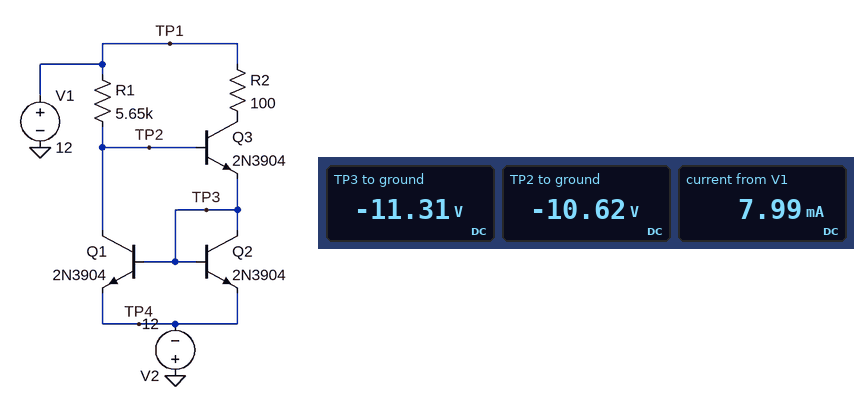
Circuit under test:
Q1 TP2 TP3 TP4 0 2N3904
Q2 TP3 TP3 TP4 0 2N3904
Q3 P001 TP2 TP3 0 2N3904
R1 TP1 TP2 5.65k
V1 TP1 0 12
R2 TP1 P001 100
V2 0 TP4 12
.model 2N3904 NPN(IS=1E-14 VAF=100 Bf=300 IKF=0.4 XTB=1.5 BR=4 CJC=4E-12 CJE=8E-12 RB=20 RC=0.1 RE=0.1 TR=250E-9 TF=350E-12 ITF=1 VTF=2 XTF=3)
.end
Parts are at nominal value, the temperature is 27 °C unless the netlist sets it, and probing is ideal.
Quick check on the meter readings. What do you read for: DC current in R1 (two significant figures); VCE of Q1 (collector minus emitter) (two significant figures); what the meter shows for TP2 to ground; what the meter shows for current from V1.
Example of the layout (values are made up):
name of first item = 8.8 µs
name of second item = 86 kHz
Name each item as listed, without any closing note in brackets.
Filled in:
DC current in R1 = 4.0 mA
VCE of Q1 (collector minus emitter) = 1.4 V
what the meter shows for TP2 to ground = -10.62 V
what the meter shows for current from V1 = 7.99 mA
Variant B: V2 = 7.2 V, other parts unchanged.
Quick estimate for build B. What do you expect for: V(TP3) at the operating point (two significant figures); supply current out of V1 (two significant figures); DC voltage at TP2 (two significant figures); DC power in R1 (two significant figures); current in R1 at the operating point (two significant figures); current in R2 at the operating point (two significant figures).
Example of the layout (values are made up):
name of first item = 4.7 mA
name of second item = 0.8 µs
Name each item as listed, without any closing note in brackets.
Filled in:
V(TP3) at the operating point = -6.5 V
supply current out of V1 = 6.3 mA
DC voltage at TP2 = -5.8 V
DC power in R1 = 56 mW
current in R1 at the operating point = 3.2 mA
current in R2 at the operating point = 3.1 mA
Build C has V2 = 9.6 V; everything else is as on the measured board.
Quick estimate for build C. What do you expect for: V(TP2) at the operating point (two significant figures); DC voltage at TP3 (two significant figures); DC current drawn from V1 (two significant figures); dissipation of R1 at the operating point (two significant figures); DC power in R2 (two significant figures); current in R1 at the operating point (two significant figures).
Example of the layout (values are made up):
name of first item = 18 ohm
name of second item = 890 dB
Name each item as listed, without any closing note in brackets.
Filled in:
V(TP2) at the operating point = -8.2 V
DC voltage at TP3 = -8.9 V
DC current drawn from V1 = 7.1 mA
dissipation of R1 at the operating point = 72 mW
DC power in R2 = 1.3 mW
current in R1 at the operating point = 3.6 mA
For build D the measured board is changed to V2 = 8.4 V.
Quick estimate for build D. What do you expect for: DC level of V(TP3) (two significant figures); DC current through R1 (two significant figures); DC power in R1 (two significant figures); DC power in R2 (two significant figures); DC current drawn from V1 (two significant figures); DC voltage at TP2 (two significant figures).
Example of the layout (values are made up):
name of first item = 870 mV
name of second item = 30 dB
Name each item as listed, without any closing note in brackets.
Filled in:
DC level of V(TP3) = -7.7 V
DC current through R1 = 3.4 mA
DC power in R1 = 64 mW
DC power in R2 = 1.1 mW
DC current drawn from V1 = 6.7 mA
DC voltage at TP2 = -7.0 V
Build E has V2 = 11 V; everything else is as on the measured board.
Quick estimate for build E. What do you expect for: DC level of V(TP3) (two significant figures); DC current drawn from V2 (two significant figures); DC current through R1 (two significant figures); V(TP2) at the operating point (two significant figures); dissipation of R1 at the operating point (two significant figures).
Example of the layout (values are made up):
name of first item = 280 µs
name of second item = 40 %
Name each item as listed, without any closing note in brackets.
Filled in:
DC level of V(TP3) = -10 V
DC current drawn from V2 = 7.6 mA
DC current through R1 = 3.8 mA
V(TP2) at the operating point = -9.6 V
dissipation of R1 at the operating point = 83 mW
